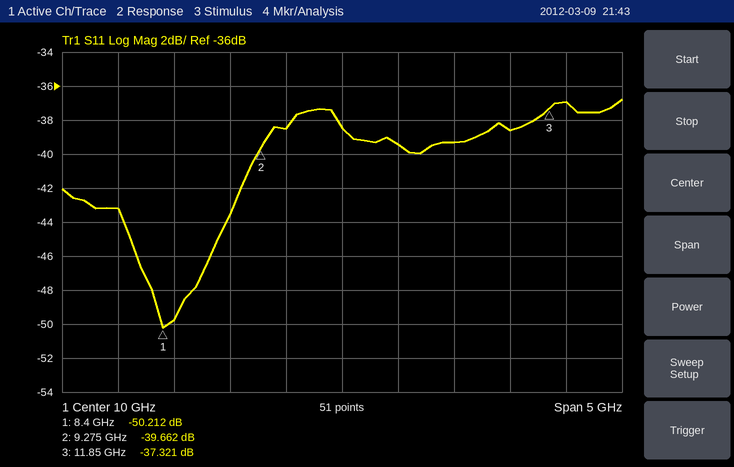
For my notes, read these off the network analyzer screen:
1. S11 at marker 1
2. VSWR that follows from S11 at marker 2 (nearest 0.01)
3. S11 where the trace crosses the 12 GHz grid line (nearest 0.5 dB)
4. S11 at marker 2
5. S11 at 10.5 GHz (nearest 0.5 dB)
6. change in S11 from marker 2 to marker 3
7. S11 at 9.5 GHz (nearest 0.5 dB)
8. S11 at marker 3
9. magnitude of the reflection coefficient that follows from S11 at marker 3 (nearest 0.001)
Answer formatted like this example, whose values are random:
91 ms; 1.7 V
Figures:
-50.212 dB; 1.02; -37.0 dB; -39.662 dB; -39.5 dB; 2.341 dB; -38.5 dB; -37.321 dB; 0.014
